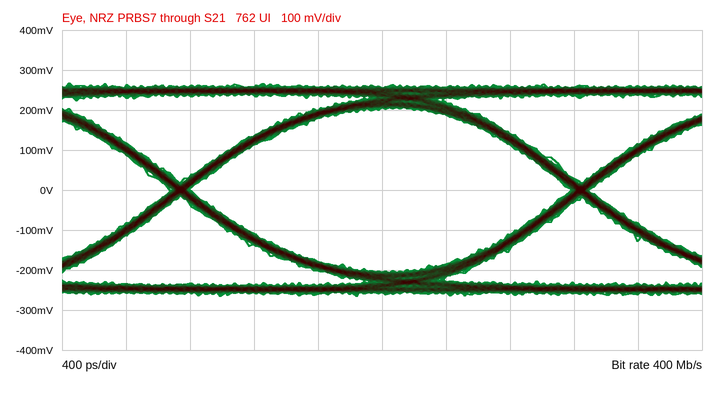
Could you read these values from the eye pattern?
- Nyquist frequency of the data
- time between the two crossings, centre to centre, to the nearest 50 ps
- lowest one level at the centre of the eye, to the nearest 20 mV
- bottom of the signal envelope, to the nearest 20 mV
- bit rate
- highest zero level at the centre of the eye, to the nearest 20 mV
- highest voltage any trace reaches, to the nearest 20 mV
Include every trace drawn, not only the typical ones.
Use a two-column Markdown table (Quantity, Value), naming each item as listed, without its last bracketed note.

| Quantity | Value |
|---|---|
| Nyquist frequency of the data | 200 MHz |
| time between the two crossings, centre to centre, to the nearest 50 ps | 2.50 ns |
| lowest one level at the centre of the eye, to the nearest 20 mV | 200 mV |
| bottom of the signal envelope, to the nearest 20 mV | -260 mV |
| bit rate | 400 Mb/s |
| highest zero level at the centre of the eye, to the nearest 20 mV | -200 mV |
| highest voltage any trace reaches, to the nearest 20 mV | 260 mV |
